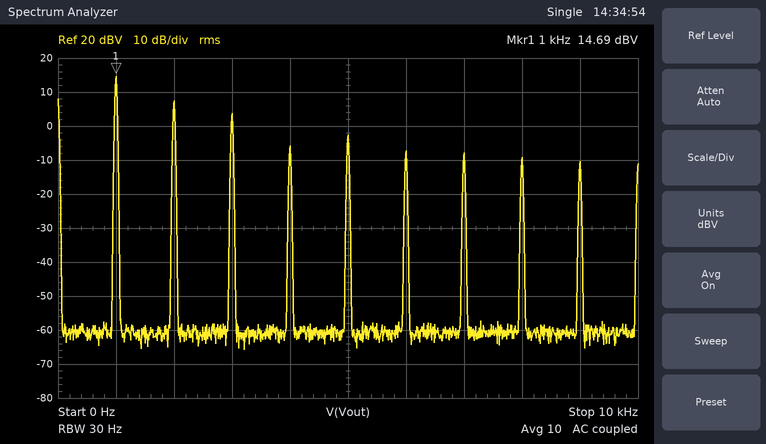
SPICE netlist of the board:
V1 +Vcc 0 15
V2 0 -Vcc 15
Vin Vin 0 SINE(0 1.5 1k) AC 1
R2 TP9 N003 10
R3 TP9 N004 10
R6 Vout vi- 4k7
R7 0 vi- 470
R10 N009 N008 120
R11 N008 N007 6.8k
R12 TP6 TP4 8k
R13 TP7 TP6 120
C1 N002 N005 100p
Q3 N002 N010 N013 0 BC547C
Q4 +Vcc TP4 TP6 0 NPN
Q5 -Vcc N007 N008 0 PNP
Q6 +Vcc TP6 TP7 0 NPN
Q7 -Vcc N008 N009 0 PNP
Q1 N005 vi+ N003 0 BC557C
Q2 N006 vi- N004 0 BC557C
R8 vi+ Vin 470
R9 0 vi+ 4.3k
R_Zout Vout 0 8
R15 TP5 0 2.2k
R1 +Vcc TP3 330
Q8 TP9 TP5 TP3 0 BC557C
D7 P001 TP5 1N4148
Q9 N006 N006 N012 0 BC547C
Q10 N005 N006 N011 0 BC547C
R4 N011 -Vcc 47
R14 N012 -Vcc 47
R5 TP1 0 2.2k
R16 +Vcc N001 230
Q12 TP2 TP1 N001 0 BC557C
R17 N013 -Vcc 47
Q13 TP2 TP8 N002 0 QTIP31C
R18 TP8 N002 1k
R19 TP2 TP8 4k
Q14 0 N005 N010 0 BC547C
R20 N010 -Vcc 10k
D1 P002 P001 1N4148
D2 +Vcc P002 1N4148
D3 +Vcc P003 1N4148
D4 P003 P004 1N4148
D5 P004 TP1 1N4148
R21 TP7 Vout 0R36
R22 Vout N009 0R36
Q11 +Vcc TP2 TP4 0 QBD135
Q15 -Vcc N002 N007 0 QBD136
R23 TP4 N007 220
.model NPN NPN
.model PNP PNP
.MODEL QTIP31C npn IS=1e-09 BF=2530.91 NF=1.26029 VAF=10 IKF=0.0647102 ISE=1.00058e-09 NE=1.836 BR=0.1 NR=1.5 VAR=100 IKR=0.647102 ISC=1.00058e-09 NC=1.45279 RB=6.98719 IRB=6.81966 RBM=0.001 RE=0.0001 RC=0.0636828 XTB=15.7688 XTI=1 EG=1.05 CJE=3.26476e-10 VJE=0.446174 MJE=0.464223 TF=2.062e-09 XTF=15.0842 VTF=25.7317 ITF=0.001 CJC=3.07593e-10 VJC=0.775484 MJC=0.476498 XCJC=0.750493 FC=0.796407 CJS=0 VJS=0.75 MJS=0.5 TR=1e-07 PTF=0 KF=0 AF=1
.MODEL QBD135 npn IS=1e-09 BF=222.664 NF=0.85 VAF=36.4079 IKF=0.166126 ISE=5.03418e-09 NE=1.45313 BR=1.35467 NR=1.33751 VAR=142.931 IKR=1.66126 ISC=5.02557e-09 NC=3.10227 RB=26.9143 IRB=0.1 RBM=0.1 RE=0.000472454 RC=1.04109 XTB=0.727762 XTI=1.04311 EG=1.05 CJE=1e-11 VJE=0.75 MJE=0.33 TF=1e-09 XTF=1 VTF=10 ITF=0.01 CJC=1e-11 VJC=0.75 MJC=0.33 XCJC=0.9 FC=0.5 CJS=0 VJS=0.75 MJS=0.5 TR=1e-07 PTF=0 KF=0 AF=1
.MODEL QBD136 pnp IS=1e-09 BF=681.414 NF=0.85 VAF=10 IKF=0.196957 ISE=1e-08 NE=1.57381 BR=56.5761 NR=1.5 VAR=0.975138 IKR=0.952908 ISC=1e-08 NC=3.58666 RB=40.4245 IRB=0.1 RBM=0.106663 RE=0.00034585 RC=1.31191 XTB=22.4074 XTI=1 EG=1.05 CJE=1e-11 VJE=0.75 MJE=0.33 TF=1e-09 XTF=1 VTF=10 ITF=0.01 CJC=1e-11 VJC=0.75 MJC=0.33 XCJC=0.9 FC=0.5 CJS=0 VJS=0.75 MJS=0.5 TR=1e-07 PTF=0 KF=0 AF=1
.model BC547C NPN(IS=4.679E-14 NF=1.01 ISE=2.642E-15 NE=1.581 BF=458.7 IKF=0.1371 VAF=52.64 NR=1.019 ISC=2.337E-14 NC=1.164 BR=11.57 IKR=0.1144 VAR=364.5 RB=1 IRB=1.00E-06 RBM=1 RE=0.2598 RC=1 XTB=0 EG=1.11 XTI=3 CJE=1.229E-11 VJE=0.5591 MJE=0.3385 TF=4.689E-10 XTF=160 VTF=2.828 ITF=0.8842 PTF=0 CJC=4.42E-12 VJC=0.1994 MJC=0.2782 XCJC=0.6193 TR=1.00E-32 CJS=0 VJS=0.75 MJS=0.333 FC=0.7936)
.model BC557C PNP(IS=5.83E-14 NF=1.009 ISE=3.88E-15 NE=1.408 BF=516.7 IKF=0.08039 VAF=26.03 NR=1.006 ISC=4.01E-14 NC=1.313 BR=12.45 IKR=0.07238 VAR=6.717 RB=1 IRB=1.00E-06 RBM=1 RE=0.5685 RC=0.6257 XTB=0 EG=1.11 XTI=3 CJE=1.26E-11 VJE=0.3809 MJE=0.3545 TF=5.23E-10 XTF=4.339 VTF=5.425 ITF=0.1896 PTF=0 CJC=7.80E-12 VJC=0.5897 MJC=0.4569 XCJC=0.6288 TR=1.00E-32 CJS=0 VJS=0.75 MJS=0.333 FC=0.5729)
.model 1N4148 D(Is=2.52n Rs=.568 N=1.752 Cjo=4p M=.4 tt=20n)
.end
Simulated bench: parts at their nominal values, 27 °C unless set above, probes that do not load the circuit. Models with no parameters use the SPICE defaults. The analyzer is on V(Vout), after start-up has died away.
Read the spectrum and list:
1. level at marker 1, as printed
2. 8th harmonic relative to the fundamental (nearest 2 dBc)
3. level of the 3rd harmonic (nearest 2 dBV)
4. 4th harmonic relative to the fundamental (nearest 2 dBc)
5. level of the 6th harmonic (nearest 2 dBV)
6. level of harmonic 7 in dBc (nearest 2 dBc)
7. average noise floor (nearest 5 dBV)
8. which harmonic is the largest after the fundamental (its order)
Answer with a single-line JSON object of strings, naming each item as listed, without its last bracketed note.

{"level at marker 1, as printed": "14.69 dBV", "8th harmonic relative to the fundamental": "-24 dBc", "level of the 3rd harmonic": "4 dBV", "4th harmonic relative to the fundamental": "-20 dBc", "level of the 6th harmonic": "-8 dBV", "level of harmonic 7 in dBc": "-22 dBc", "average noise floor": "-60 dBV", "which harmonic is the largest after the fundamental": "2"}
